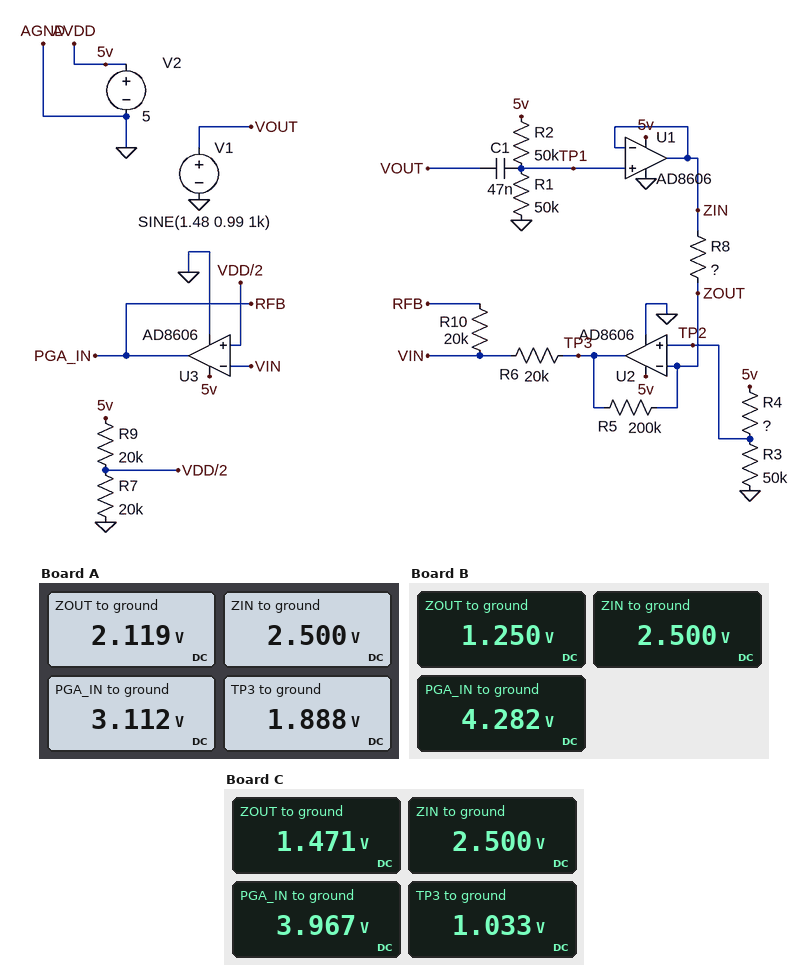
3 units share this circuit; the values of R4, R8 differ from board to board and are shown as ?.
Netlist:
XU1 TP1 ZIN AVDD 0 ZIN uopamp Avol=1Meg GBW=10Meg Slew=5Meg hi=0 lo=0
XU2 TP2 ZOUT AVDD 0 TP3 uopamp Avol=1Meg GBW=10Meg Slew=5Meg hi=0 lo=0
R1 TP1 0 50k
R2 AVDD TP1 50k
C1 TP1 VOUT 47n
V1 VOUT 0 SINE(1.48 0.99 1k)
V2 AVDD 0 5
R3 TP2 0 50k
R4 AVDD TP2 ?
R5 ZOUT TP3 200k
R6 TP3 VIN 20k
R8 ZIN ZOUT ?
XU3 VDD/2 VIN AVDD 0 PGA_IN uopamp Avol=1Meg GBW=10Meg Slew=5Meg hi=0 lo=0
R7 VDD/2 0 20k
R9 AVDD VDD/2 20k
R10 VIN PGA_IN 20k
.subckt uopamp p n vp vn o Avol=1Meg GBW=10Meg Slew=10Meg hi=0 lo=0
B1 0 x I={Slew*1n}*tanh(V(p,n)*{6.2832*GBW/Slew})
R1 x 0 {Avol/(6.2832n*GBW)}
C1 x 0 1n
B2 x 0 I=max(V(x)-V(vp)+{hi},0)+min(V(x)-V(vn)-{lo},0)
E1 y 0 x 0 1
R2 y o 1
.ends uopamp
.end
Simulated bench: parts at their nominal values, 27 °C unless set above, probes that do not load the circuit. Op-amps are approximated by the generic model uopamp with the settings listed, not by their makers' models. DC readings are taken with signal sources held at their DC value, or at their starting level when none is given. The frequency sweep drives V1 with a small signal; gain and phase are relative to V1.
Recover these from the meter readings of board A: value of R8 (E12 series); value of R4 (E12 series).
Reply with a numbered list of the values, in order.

1. 330 kΩ
2. 68 kΩ
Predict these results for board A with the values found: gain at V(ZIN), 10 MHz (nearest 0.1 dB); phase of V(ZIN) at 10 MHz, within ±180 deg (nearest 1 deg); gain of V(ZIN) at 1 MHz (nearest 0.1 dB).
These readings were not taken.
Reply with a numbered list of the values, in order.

1. -3.0 dB
2. -45 deg
3. 0 dB
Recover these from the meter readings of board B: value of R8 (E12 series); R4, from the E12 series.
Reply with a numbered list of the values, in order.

1. 470 kΩ
2. 150 kΩ
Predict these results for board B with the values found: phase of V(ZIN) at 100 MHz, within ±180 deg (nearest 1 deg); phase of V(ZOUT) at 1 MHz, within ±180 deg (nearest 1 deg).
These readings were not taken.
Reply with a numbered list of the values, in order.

1. -84 deg
2. 76 deg
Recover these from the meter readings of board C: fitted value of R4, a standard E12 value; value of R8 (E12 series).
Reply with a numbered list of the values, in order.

1. 120 kΩ
2. 470 kΩ
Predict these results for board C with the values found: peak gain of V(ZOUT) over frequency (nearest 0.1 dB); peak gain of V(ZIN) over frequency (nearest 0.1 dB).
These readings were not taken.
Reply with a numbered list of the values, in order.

1. -15.1 dB
2. 0 dB
